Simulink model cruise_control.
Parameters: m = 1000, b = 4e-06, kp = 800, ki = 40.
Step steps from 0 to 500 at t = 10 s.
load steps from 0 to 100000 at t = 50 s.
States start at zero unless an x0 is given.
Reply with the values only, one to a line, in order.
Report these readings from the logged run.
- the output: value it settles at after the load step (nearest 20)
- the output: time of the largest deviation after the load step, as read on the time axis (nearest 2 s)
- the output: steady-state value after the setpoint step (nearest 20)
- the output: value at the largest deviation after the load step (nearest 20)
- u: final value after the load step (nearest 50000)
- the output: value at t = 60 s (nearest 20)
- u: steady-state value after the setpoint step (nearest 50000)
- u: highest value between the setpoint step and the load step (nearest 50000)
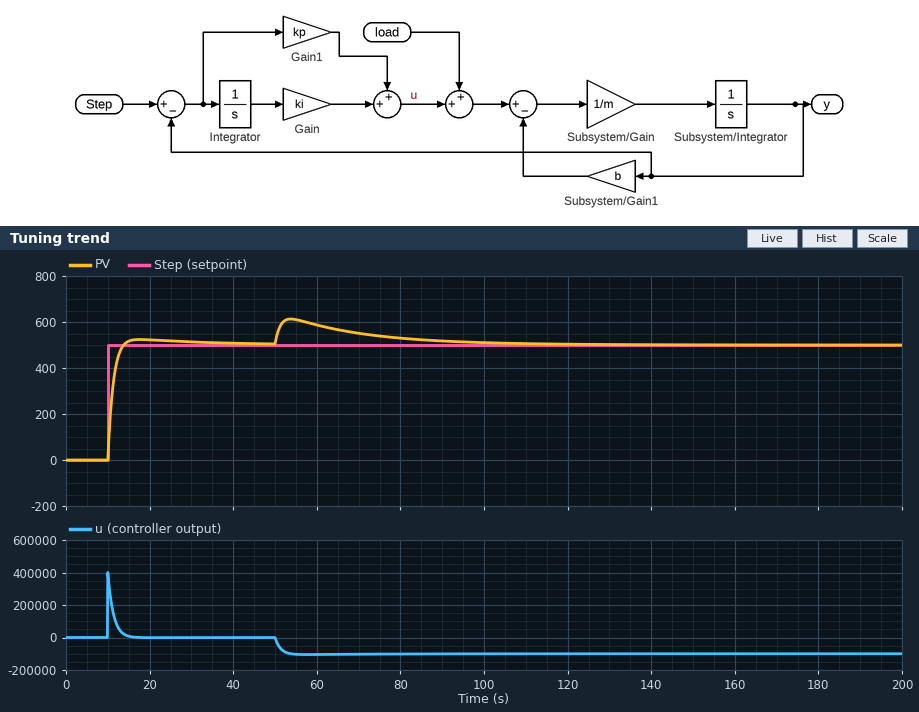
500
54 s
500
620
-100000
580
0
400000
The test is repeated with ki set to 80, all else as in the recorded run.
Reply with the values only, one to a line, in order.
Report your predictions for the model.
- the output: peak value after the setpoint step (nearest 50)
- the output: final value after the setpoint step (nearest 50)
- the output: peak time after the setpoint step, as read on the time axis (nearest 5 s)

550
500
15 s
